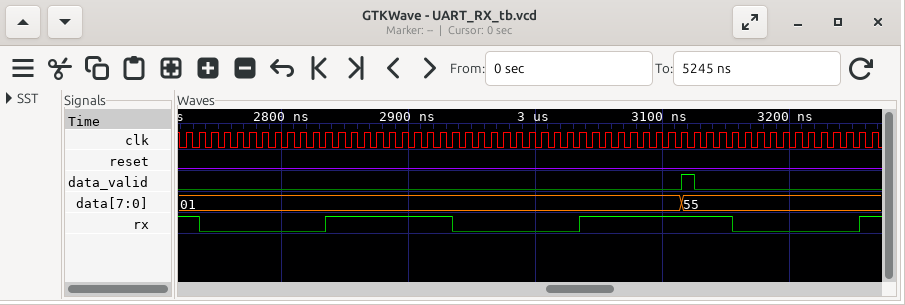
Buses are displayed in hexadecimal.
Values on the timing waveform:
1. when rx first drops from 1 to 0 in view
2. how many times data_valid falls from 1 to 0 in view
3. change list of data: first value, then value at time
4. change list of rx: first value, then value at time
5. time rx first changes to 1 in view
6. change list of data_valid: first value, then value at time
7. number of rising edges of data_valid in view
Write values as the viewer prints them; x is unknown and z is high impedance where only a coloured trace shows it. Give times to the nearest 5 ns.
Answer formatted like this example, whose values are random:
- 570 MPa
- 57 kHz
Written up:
- 2735 ns
- 1
- 01, 55 at 3115 ns
- 1, 0 at 2735 ns, 1 at 2835 ns, 0 at 2935 ns, 1 at 3035 ns, 0 at 3155 ns, 1 at 3255 ns
- 2835 ns
- 0, 1 at 3115 ns, 0 at 3125 ns
- 1
